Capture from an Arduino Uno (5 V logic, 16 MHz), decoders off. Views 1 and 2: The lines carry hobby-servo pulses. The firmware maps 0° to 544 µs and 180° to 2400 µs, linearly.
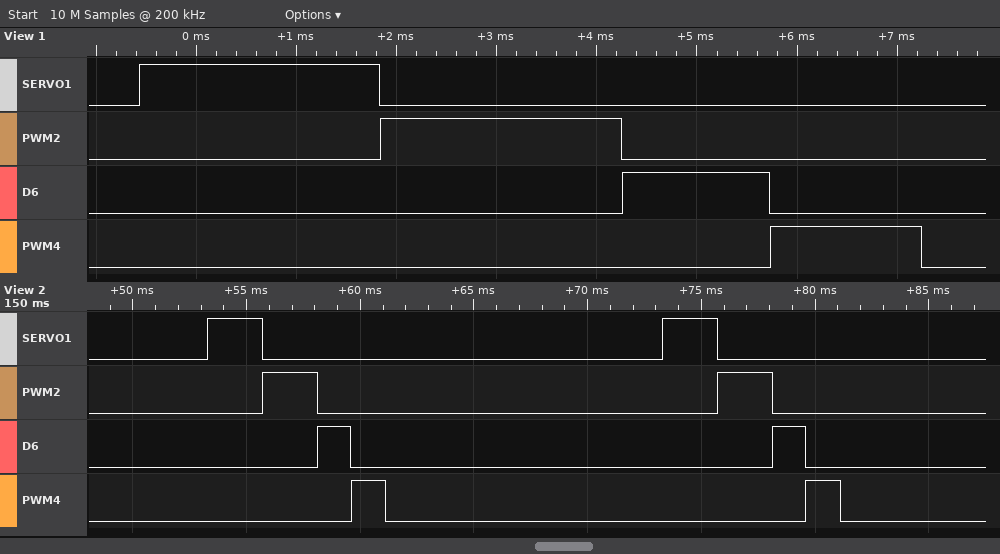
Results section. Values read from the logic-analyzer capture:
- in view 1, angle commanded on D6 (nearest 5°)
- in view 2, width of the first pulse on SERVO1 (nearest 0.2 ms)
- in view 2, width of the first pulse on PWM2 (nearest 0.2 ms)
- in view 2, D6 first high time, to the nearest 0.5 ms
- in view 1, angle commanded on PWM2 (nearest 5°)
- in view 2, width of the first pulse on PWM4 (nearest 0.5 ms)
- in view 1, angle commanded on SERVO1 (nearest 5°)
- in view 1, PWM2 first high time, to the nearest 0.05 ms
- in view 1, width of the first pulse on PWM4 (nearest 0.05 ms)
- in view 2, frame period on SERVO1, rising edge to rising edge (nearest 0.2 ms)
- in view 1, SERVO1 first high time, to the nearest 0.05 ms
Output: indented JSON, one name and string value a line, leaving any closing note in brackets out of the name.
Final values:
{
  "in view 1, angle commanded on D6": "90°",
  "in view 2, width of the first pulse on SERVO1": "2.4 ms",
  "in view 2, width of the first pulse on PWM2": "2.4 ms",
  "in view 2, D6 first high time, to the nearest 0.5 ms": "1.5 ms",
  "in view 1, angle commanded on PWM2": "180°",
  "in view 2, width of the first pulse on PWM4": "1.5 ms",
  "in view 1, angle commanded on SERVO1": "180°",
  "in view 1, PWM2 first high time, to the nearest 0.05 ms": "2.40 ms",
  "in view 1, width of the first pulse on PWM4": "1.50 ms",
  "in view 2, frame period on SERVO1, rising edge to rising edge": "20.0 ms",
  "in view 1, SERVO1 first high time, to the nearest 0.05 ms": "2.40 ms"
}
